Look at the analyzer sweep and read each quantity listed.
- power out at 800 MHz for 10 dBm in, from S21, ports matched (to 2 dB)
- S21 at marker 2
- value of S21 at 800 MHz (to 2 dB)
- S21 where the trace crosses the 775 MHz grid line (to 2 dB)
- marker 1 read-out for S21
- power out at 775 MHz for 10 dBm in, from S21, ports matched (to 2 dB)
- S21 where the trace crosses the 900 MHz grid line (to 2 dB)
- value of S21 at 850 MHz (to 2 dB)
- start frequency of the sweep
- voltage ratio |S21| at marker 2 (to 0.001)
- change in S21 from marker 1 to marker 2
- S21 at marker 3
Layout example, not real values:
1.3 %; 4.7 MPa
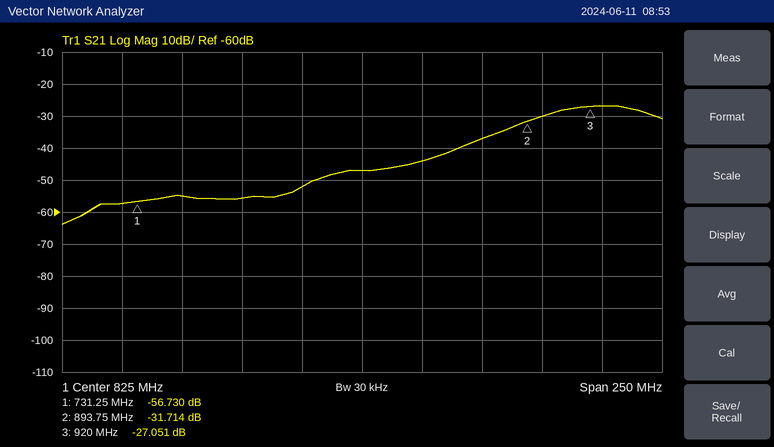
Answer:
-42 dBm; -31.714 dB; -52 dB; -56 dB; -56.730 dB; -46 dBm; -30 dB; -44 dB; 700 MHz; 0.026; 25.016 dB; -27.051 dB
